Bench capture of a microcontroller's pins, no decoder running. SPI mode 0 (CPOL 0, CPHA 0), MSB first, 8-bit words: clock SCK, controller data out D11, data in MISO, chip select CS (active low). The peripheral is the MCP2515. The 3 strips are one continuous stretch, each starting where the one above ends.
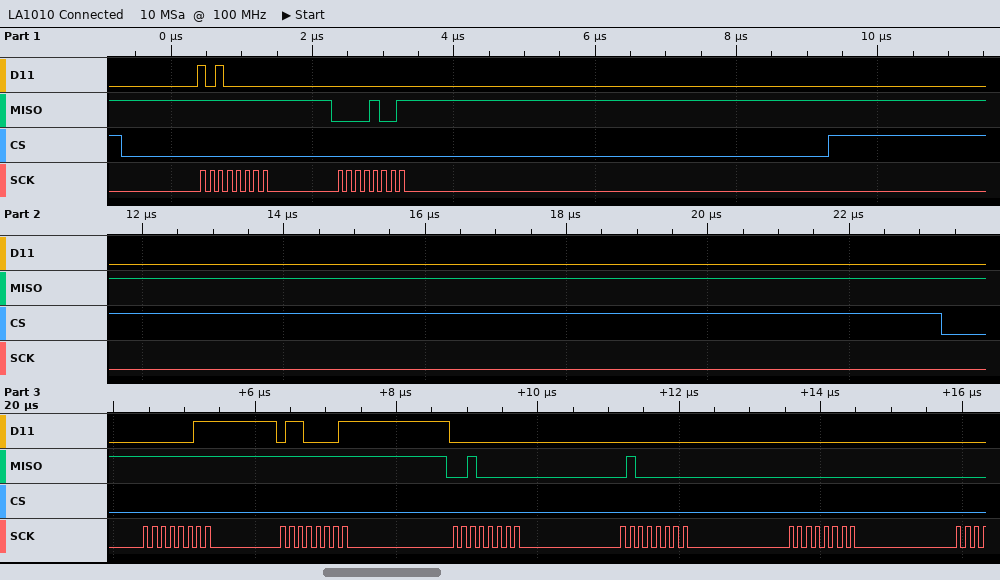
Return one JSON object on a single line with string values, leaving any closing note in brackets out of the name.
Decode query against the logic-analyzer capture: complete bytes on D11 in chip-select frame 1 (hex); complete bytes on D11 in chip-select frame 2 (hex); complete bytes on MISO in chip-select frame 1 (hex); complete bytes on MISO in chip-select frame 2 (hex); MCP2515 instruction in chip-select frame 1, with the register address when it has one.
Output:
{"complete bytes on D11 in chip-select frame 1": "A0 00", "complete bytes on D11 in chip-select frame 2": "03 61 00 00 00", "complete bytes on MISO in chip-select frame 1": "FF 09", "complete bytes on MISO in chip-select frame 2": "FF FF 20 40 00", "MCP2515 instruction in chip-select frame 1, with the register address when it has one": "READ STATUS"}
